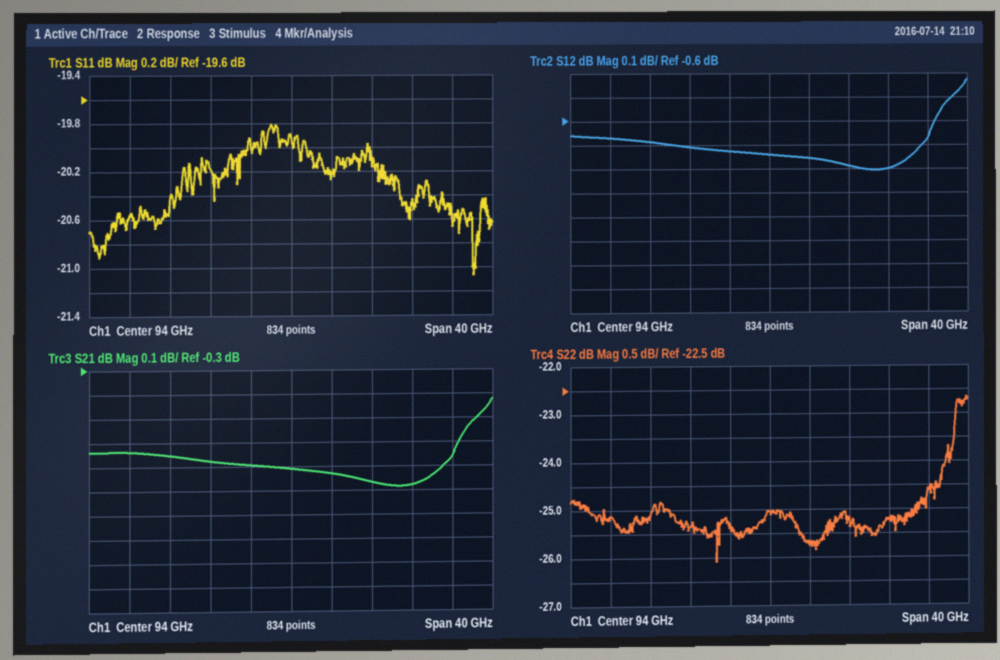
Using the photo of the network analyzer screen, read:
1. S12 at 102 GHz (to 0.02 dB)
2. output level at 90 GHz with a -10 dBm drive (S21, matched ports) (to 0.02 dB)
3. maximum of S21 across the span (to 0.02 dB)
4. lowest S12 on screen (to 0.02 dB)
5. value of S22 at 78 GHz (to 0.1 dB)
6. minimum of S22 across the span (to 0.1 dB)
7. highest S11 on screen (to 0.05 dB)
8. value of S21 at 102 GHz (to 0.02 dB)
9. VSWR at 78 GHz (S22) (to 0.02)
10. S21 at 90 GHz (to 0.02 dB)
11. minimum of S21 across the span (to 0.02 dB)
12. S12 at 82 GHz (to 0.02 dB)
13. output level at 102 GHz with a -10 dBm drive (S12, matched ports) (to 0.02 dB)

-0.78 dB
-10.70 dBm
-0.42 dB
-0.80 dB
-25.1 dB
-26.1 dB
-19.80 dB
-0.76 dB
1.12
-0.70 dB
-0.78 dB
-0.68 dB
-10.78 dBm
